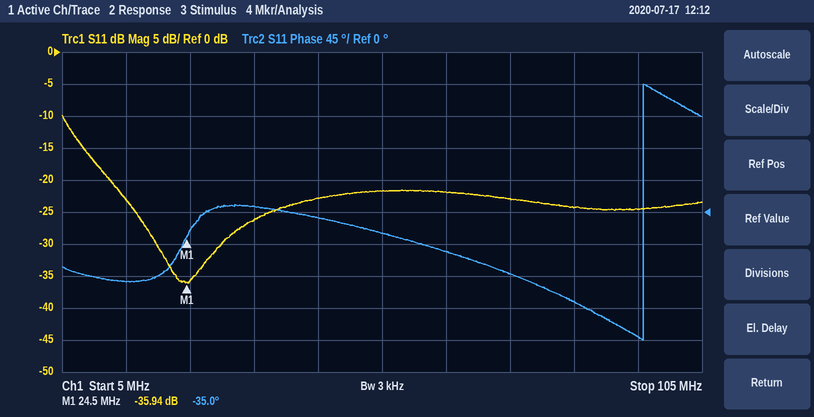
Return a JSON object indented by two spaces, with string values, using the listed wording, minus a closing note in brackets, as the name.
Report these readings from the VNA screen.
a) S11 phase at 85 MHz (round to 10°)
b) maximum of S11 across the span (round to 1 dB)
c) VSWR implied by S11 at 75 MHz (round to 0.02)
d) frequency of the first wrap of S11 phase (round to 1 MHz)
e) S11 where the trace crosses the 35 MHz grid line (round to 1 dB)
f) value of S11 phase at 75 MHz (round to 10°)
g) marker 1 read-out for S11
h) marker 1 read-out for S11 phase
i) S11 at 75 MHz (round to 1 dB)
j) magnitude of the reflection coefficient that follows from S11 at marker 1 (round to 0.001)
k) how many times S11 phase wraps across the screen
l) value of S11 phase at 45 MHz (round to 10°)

{
  "S11 phase at 85 MHz": "-130°",
  "maximum of S11 across the span": "-10 dB",
  "VSWR implied by S11 at 75 MHz": "1.16",
  "frequency of the first wrap of S11 phase": "96 MHz",
  "S11 where the trace crosses the 35 MHz grid line": "-26 dB",
  "value of S11 phase at 75 MHz": "-90°",
  "marker 1 read-out for S11": "-35.94 dB",
  "marker 1 read-out for S11 phase": "-35.0°",
  "S11 at 75 MHz": "-23 dB",
  "magnitude of the reflection coefficient that follows from S11 at marker 1": "0.016",
  "how many times S11 phase wraps across the screen": "1",
  "value of S11 phase at 45 MHz": "-10°"
}
